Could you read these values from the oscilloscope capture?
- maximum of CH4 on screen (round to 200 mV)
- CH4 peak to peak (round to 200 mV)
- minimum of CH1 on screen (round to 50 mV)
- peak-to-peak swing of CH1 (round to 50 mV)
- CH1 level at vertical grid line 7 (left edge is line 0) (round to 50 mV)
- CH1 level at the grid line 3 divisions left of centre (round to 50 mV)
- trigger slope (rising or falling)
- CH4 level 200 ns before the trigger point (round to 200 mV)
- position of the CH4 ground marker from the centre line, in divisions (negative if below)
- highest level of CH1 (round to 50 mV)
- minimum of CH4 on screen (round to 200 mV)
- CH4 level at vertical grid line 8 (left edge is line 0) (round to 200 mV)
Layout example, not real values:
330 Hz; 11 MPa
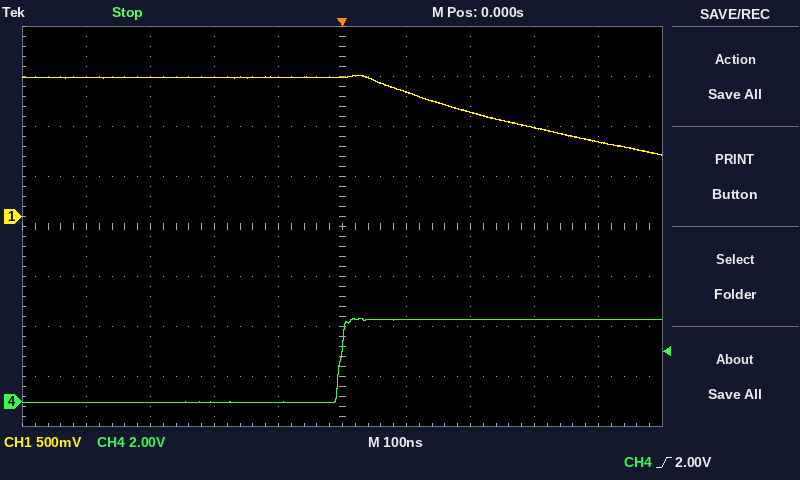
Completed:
3.4 V; 3.4 V; 600 mV; 800 mV; 1.05 V; 1.40 V; rising; 0.0 V; -3.5 div; 1.40 V; 0.0 V; 3.2 V
